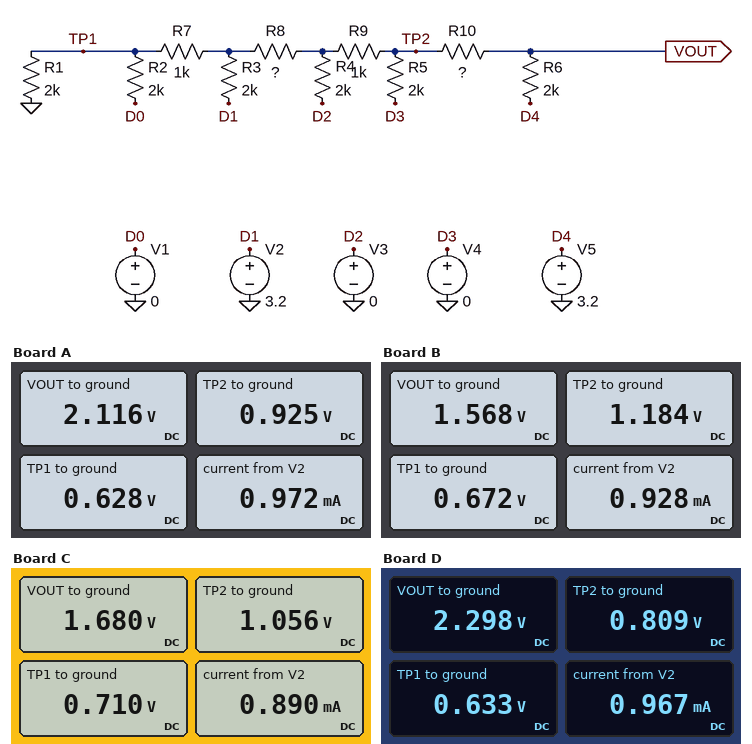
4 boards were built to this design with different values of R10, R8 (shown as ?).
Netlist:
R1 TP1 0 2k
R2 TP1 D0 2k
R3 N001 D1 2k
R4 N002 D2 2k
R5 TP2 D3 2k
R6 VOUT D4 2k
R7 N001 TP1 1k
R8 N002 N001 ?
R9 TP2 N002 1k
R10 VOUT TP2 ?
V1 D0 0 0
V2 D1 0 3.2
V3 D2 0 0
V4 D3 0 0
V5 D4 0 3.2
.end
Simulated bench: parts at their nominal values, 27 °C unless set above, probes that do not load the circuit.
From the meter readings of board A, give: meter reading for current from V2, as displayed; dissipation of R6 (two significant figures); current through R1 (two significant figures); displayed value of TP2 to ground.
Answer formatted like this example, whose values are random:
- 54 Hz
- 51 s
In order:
- 0.972 mA
- 590 µW
- 310 µA
- 0.925 V
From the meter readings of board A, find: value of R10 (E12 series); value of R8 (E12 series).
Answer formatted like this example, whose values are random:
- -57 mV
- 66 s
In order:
- 2.2 kΩ
- 1.2 kΩ
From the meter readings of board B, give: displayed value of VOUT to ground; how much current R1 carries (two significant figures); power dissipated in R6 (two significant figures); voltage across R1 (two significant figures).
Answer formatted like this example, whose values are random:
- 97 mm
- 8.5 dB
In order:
- 1.568 V
- 340 µA
- 1.3 mW
- 670 mV
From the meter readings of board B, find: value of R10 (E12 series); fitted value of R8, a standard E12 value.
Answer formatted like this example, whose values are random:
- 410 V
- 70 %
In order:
- 470 Ω
- 1.5 kΩ
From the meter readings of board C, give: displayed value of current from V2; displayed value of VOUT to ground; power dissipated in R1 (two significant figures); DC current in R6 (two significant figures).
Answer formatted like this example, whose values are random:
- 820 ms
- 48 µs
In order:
- 0.890 mA
- 1.680 V
- 250 µW
- 760 µA
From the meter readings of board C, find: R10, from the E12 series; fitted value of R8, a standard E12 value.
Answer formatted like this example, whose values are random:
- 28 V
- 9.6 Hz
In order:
- 820 Ω
- 3.3 kΩ
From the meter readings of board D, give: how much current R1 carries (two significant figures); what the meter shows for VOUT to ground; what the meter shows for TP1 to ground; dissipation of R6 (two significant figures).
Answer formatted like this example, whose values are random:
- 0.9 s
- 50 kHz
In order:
- 320 µA
- 2.298 V
- 0.633 V
- 410 µW
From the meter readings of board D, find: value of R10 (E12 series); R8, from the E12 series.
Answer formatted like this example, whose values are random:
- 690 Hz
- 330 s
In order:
- 3.3 kΩ
- 1.5 kΩ
